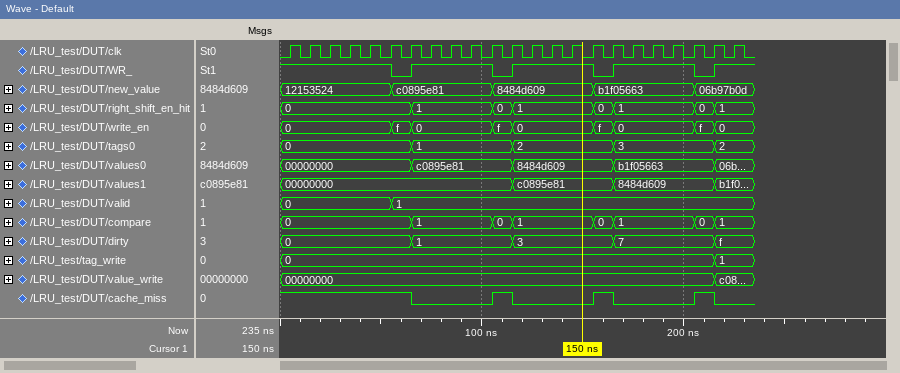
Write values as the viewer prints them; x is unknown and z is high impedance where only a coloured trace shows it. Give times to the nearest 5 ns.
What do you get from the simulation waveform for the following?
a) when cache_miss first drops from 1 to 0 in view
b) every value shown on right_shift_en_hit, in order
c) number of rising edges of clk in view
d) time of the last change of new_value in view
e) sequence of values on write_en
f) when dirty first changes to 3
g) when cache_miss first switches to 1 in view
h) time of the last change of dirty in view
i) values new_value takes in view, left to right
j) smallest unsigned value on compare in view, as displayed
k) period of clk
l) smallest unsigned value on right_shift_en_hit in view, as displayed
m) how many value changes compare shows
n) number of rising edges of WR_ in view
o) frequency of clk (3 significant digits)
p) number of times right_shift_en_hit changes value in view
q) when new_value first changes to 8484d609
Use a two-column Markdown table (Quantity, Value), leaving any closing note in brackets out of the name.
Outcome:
| Quantity | Value |
|---|---|
| when cache_miss first drops from 1 to 0 in view | 65 ns |
| every value shown on right_shift_en_hit, in order | 0, 1, 0, 1, 0, 1, 0, 1 |
| number of rising edges of clk in view | 23 |
| time of the last change of new_value in view | 205 ns |
| sequence of values on write_en | 0, f, 0, f, 0, f, 0, f, 0 |
| when dirty first changes to 3 | 115 ns |
| when cache_miss first switches to 1 in view | 105 ns |
| time of the last change of dirty in view | 215 ns |
| values new_value takes in view, left to right | 12153524, c0895e81, 8484d609, b1f05663, 06b97b0d |
| smallest unsigned value on compare in view, as displayed | 0 |
| period of clk | 10 ns |
| smallest unsigned value on right_shift_en_hit in view, as displayed | 0 |
| how many value changes compare shows | 7 |
| number of rising edges of WR_ in view | 4 |
| frequency of clk | 100 MHz |
| number of times right_shift_en_hit changes value in view | 7 |
| when new_value first changes to 8484d609 | 105 ns |
